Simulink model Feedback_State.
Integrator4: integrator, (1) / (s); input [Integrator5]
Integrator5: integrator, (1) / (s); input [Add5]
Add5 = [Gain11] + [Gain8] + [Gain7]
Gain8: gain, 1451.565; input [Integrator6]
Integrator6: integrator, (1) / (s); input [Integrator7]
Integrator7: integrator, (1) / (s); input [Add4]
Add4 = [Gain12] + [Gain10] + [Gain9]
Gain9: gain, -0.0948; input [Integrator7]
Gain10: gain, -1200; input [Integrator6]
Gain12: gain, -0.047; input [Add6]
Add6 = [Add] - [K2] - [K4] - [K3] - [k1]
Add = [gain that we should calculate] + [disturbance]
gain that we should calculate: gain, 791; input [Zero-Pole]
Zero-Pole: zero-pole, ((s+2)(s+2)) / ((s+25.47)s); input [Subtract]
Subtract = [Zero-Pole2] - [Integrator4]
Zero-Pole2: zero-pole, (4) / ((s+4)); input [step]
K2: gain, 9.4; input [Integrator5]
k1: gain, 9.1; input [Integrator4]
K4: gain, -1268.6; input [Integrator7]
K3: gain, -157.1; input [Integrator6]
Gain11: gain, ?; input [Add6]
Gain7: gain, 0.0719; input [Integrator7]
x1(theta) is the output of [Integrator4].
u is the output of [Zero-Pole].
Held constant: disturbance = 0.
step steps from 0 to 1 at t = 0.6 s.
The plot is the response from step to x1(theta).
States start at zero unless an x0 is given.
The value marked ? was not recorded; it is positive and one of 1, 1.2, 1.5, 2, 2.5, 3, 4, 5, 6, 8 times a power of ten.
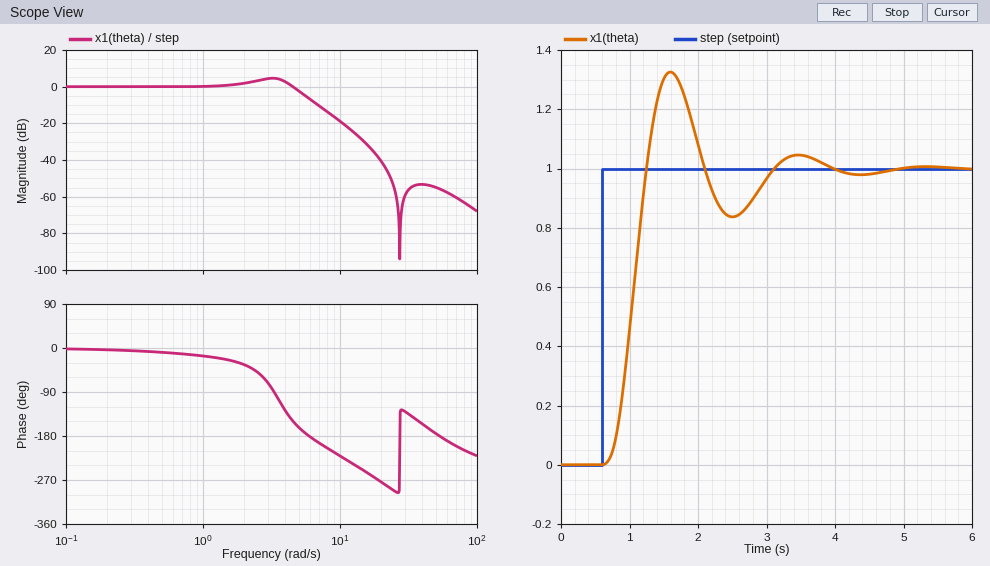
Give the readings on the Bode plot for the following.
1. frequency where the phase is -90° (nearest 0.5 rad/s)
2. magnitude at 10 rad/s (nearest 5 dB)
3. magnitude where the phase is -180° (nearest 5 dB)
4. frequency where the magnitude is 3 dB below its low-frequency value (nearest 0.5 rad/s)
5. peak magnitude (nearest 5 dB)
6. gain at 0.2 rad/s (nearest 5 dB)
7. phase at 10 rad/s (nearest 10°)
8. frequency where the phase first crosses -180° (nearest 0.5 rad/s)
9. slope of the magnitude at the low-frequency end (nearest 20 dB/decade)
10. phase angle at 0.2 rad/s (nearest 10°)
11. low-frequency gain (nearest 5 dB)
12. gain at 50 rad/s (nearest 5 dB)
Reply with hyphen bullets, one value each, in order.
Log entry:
- 3.5 rad/s
- -20 dB
- -5 dB
- 5.0 rad/s
- 5 dB
- 0 dB
- -220°
- 6.0 rad/s
- 0 dB/decade
- 0°
- 0 dB
- -55 dB
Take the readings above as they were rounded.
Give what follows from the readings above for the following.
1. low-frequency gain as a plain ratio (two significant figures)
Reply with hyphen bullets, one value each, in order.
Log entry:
- 1.0
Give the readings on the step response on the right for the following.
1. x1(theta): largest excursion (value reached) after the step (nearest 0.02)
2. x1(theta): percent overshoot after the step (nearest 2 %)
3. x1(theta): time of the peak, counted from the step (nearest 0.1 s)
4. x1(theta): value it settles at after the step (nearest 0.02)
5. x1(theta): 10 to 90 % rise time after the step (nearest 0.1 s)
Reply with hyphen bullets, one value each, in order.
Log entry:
- 1.32
- 32 %
- 1.0 s
- 1.00
- 0.4 s
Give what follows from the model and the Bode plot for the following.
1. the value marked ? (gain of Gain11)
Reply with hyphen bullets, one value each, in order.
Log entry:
- 0.15
